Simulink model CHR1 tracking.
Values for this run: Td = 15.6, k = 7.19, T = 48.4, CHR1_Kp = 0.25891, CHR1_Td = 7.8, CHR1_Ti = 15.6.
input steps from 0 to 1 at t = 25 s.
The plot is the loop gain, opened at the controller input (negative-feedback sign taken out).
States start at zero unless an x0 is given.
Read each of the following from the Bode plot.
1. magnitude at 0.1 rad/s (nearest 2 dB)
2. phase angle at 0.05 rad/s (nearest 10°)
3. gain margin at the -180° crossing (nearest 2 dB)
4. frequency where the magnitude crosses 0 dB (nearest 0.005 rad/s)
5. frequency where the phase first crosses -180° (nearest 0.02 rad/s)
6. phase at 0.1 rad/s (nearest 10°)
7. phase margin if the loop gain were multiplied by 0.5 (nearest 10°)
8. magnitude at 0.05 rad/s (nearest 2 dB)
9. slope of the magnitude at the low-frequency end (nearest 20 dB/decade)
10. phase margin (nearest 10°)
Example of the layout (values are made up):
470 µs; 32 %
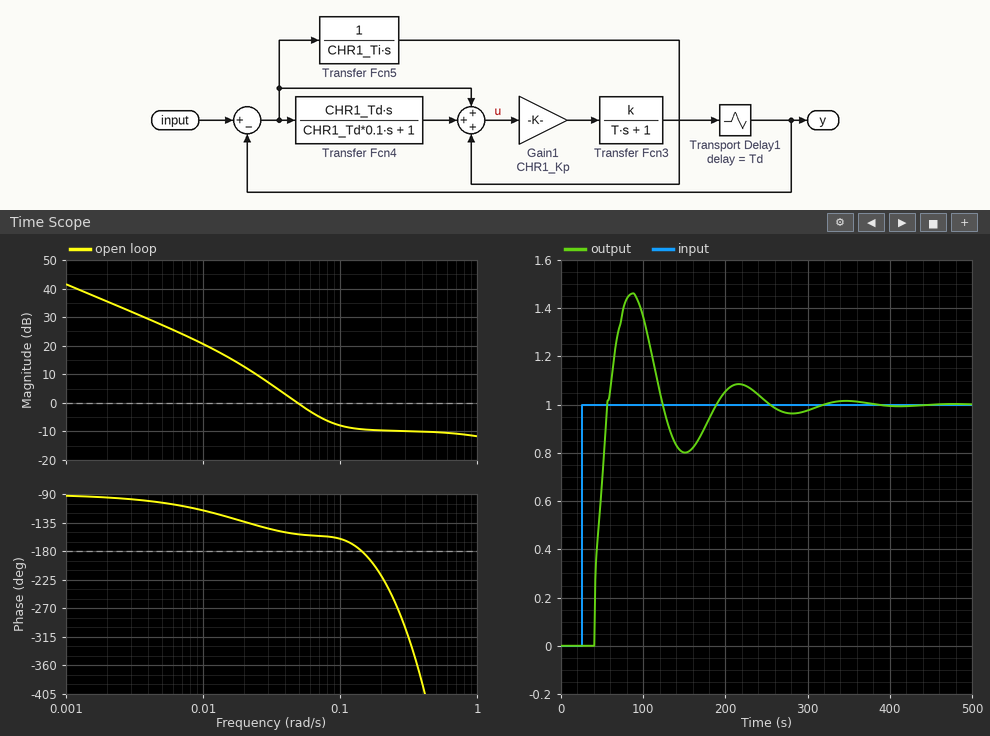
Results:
-8 dB; -150°; 10 dB; 0.050 rad/s; 0.14 rad/s; -160°; 30°; 0 dB; -20 dB/decade; 30°
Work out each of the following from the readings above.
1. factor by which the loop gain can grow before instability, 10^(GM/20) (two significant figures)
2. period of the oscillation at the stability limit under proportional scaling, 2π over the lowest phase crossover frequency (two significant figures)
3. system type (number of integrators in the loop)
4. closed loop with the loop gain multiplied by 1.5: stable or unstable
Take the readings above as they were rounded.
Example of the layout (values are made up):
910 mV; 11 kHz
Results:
3.2; 45 s; 1; stable
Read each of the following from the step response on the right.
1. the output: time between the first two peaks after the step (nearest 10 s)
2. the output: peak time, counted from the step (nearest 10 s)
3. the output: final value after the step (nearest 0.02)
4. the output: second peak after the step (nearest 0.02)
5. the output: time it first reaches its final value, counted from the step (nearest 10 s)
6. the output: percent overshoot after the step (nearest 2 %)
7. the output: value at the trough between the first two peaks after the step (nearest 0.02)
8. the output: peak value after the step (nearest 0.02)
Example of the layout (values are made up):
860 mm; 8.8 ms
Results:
130 s; 60 s; 1.00; 1.08; 30 s; 46 %; 0.80; 1.46
